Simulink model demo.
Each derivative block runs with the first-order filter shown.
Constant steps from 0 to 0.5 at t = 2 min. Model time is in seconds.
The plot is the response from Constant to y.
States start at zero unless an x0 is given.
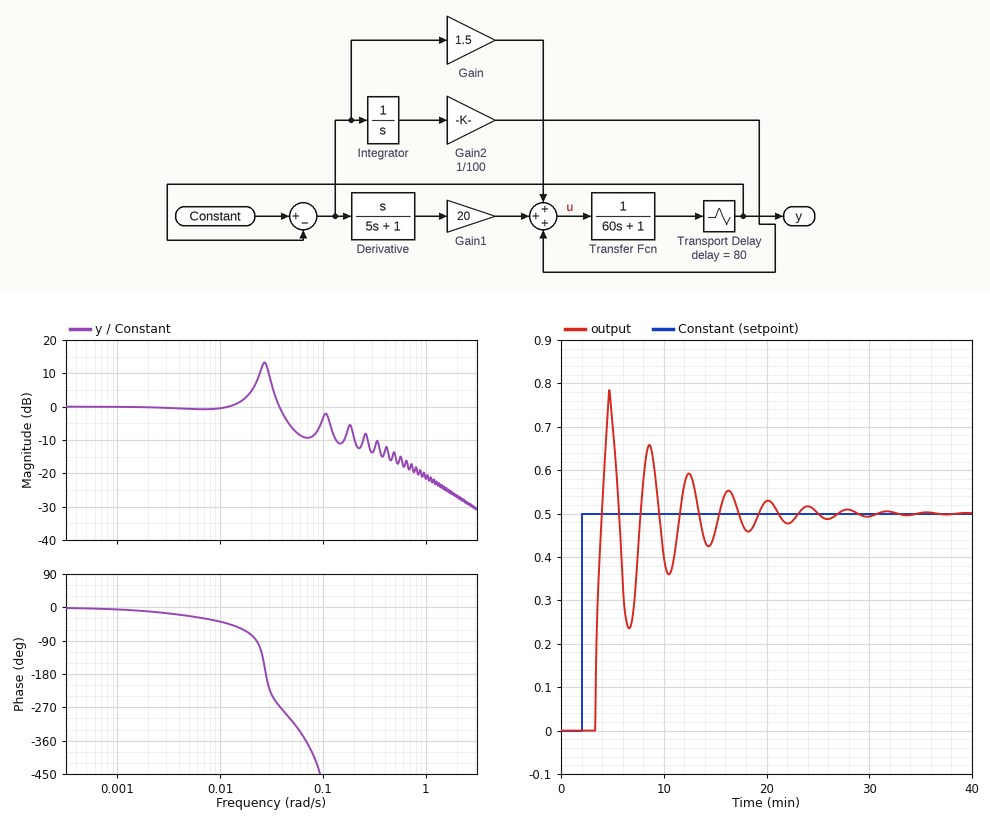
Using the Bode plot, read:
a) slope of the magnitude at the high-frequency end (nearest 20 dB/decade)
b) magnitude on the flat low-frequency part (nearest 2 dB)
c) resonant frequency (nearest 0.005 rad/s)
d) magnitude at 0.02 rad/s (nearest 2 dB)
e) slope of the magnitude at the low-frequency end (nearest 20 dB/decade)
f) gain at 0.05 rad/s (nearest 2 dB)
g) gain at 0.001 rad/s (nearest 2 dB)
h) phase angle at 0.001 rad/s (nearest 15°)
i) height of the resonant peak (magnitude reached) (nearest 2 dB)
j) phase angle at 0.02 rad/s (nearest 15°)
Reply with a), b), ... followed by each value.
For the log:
a) -20 dB/decade
b) 0 dB
c) 0.025 rad/s
d) 4 dB
e) 0 dB/decade
f) -6 dB
g) 0 dB
h) 0°
i) 14 dB
j) -75°
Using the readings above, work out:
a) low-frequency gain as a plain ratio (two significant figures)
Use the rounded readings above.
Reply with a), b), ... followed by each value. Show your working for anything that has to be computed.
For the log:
a) 10^(0 / 20) = 1.0
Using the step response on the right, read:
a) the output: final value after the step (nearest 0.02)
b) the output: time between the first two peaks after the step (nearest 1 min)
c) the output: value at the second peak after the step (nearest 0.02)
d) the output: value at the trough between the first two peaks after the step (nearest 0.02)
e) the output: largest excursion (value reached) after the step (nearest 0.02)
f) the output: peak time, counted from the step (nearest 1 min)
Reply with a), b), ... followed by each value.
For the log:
a) 0.50
b) 4 min
c) 0.66
d) 0.24
e) 0.78
f) 3 min
